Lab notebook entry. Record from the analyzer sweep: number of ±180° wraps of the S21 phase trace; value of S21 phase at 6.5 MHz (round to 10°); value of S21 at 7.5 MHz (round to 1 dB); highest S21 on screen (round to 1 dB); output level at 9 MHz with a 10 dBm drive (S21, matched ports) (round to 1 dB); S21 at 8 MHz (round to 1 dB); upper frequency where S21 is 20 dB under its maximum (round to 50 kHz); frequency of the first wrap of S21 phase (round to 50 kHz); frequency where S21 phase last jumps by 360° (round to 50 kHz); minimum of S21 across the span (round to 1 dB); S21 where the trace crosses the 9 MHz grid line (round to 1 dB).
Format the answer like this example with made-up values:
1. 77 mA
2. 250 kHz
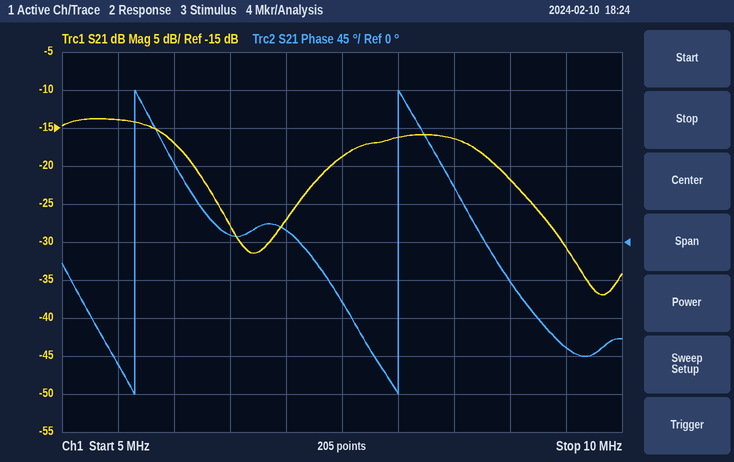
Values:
1. 2
2. 10°
3. -19 dB
4. -14 dB
5. -12 dBm
6. -16 dB
7. 9.65 MHz
8. 5.65 MHz
9. 8.00 MHz
10. -37 dB
11. -22 dB
